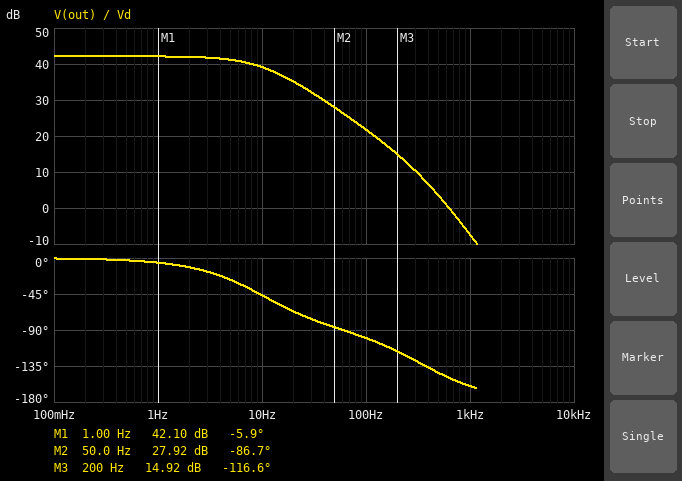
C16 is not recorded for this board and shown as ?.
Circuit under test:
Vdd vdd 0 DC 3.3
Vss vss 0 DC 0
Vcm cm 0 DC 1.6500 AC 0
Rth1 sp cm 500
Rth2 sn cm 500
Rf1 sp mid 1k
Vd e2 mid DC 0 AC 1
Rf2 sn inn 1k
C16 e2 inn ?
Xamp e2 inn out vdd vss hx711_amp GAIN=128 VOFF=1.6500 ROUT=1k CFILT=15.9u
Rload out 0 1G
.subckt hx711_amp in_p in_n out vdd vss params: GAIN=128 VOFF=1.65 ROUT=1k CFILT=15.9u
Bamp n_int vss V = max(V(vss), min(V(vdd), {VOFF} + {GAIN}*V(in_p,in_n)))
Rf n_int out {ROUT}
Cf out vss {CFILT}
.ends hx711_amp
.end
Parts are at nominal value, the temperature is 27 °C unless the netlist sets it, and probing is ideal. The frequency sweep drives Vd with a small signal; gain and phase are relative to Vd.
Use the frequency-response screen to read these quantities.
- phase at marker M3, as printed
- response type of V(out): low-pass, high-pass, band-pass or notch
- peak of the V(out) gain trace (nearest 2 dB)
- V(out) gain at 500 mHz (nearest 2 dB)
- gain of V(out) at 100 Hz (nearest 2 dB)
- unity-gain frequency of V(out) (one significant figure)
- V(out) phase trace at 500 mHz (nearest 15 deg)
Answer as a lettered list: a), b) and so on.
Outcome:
a) -116.6 deg
b) low-pass
c) 42 dB
d) 42 dB
e) 22 dB
f) 600 Hz
g) 0 deg
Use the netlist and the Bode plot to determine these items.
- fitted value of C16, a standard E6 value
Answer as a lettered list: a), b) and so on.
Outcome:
a) 150 nF
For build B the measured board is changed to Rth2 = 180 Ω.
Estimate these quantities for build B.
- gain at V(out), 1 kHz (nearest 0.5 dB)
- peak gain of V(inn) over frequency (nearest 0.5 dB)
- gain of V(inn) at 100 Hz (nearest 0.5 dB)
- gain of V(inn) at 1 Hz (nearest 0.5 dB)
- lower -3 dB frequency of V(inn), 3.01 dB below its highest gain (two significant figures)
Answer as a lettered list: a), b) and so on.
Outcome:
a) -6.5 dB
b) -7.0 dB
c) -19.5 dB
d) -59.0 dB
e) 400 Hz
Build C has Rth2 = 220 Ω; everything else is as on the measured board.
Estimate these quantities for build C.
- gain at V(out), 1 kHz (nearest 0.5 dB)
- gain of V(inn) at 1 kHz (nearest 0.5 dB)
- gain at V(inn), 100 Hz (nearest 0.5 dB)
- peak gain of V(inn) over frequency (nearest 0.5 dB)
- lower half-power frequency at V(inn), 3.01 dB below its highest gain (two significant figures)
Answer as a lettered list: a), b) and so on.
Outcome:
a) -6.5 dB
b) -7.5 dB
c) -19.0 dB
d) -7.0 dB
e) 390 Hz
